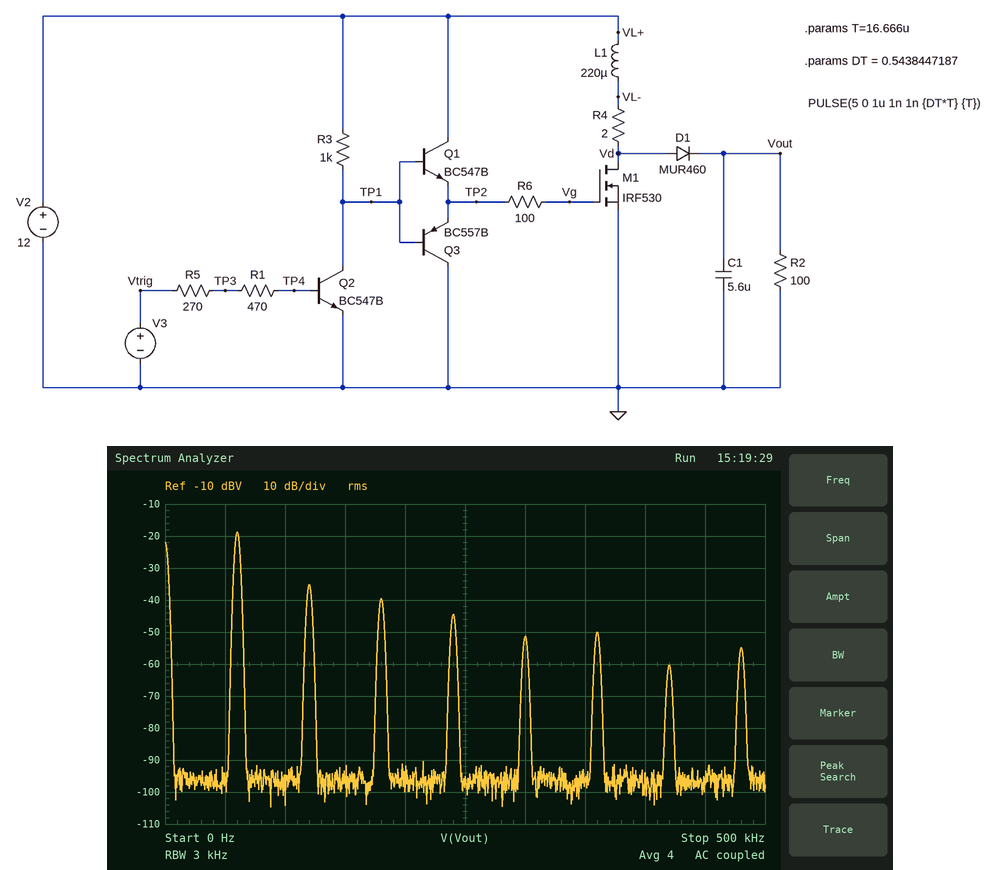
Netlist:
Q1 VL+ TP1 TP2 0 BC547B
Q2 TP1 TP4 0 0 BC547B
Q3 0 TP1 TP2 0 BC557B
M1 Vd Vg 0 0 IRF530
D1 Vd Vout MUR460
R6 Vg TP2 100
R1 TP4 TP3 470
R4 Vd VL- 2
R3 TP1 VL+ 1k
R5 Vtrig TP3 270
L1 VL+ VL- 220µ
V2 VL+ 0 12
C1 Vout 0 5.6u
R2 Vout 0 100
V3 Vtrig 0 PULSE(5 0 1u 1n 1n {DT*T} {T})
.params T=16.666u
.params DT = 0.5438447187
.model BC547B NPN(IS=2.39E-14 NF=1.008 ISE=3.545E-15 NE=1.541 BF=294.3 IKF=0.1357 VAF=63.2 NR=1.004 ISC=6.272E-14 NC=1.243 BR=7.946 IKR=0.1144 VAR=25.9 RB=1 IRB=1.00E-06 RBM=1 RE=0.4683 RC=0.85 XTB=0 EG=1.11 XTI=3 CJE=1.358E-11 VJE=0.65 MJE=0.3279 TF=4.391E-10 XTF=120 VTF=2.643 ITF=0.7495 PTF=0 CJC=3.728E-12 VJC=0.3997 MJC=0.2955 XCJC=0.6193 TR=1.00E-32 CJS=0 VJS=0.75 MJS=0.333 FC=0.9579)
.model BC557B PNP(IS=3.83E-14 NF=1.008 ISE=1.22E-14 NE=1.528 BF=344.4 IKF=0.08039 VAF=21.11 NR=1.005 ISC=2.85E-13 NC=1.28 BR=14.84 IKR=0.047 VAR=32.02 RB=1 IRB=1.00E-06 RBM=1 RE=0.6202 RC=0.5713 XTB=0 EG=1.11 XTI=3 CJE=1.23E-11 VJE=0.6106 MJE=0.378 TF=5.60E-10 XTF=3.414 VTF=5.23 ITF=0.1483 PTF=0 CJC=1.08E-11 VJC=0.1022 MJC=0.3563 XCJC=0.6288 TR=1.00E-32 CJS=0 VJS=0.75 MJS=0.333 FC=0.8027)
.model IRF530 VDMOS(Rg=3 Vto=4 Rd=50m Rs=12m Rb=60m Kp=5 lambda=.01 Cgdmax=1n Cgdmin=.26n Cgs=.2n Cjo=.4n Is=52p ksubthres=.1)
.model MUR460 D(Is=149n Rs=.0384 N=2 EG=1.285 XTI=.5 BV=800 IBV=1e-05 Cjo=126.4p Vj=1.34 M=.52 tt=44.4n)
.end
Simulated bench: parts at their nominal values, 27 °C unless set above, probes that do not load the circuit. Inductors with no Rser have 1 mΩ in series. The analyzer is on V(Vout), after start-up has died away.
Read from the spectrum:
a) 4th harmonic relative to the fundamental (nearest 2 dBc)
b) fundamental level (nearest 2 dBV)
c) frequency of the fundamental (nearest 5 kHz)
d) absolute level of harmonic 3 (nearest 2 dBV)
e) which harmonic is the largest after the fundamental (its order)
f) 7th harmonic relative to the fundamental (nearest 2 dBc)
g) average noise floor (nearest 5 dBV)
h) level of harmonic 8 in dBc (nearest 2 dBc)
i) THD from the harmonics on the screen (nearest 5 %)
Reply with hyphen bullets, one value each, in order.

- -26 dBc
- -18 dBV
- 60 kHz
- -40 dBV
- 2
- -42 dBc
- -95 dBV
- -36 dBc
- 20 %
